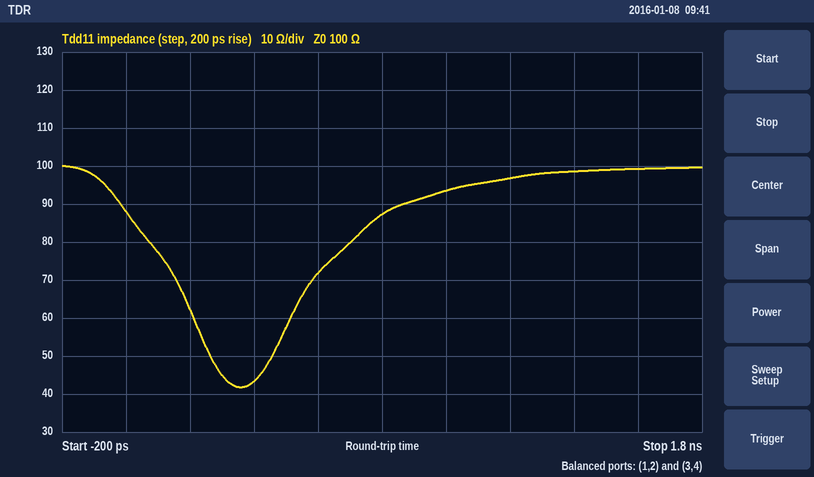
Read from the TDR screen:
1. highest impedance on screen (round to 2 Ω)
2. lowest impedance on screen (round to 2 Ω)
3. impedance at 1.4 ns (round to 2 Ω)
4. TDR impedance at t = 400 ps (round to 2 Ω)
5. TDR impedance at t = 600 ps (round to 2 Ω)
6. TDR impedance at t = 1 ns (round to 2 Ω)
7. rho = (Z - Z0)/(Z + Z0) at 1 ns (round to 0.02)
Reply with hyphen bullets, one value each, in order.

- 100 Ω
- 42 Ω
- 98 Ω
- 44 Ω
- 72 Ω
- 94 Ω
- -0.04
